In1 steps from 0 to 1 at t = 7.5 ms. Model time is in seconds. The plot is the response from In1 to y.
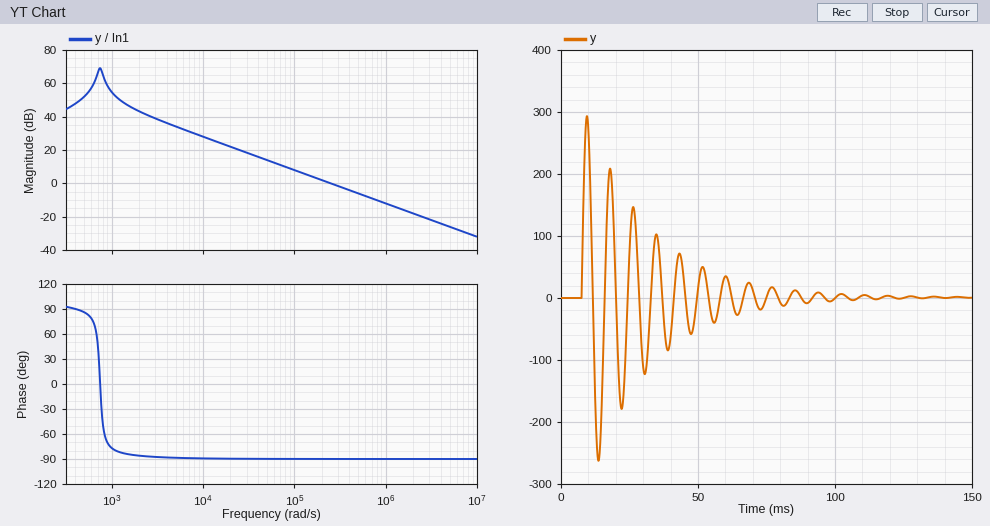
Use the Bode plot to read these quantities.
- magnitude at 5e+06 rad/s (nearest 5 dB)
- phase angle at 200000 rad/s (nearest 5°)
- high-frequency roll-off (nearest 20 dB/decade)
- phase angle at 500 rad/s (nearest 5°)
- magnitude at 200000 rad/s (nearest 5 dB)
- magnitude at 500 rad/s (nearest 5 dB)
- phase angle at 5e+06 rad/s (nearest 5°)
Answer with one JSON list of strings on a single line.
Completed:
["-25 dB", "-90°", "-20 dB/decade", "85°", "0 dB", "50 dB", "-90°"]
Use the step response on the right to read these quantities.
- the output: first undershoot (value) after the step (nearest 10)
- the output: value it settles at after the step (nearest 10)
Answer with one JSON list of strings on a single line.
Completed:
["-260", "0"]
